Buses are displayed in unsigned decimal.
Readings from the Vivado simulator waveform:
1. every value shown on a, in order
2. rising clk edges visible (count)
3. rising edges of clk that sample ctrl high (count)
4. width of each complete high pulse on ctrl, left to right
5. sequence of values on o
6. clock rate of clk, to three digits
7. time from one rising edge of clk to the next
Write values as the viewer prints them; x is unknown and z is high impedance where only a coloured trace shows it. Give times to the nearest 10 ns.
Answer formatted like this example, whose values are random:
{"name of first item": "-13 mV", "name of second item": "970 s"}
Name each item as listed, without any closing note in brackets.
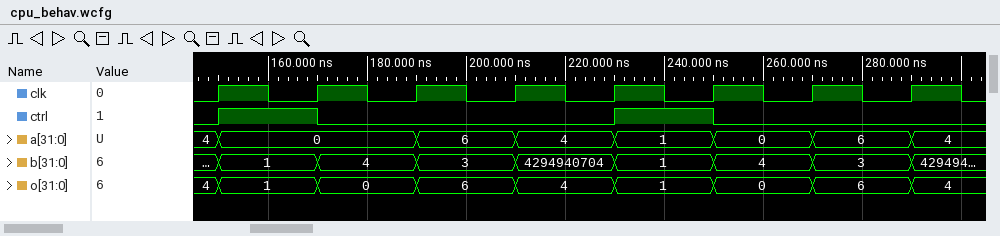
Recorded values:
{"every value shown on a, in order": "4, 0, 6, 4, 1, 0, 6, 4", "rising clk edges visible": "8", "rising edges of clk that sample ctrl high": "2", "width of each complete high pulse on ctrl, left to right": "20 ns, 20 ns", "sequence of values on o": "4, 1, 0, 6, 4, 1, 0, 6, 4", "clock rate of clk, to three digits": "50.0 MHz", "time from one rising edge of clk to the next": "20 ns"}
